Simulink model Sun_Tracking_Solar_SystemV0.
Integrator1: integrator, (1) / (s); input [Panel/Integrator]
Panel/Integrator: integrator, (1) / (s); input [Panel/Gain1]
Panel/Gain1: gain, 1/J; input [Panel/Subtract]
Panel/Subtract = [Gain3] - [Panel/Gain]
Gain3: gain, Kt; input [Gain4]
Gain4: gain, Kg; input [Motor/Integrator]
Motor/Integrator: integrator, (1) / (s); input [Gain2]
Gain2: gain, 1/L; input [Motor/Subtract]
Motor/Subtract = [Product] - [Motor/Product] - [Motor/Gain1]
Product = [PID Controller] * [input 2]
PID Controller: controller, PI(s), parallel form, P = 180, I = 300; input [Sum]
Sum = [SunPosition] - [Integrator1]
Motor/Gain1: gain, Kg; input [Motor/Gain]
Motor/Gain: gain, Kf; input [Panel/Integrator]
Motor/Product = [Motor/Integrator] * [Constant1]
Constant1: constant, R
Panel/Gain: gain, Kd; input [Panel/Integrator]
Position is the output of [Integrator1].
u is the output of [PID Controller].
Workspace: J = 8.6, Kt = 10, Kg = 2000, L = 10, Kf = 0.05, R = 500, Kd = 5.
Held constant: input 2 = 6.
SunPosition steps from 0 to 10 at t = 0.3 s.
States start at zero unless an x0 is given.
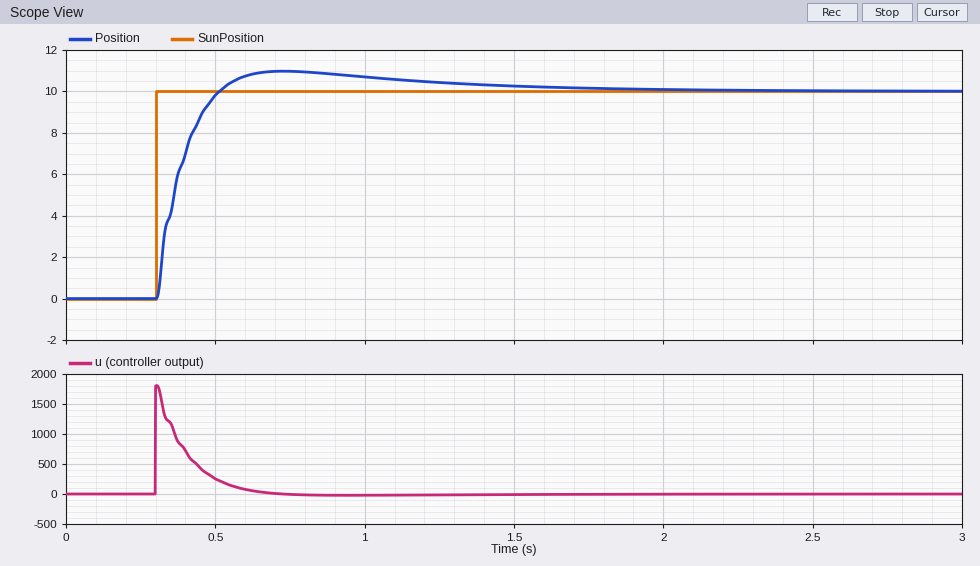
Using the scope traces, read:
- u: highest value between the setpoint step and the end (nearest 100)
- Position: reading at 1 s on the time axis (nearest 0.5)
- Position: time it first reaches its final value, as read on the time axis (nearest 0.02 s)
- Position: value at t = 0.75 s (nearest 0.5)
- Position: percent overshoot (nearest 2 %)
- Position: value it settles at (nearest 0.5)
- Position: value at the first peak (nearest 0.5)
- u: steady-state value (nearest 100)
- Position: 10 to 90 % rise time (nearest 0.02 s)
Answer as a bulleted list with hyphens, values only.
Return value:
- 1800
- 10.5
- 0.52 s
- 11.0
- 10 %
- 10.0
- 11.0
- 0
- 0.14 s
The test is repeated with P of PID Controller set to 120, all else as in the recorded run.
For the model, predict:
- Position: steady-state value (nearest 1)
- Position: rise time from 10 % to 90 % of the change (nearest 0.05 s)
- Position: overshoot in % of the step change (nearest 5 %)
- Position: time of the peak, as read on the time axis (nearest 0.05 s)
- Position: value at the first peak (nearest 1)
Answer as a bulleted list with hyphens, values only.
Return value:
- 10
- 0.20 s
- 15 %
- 0.80 s
- 12
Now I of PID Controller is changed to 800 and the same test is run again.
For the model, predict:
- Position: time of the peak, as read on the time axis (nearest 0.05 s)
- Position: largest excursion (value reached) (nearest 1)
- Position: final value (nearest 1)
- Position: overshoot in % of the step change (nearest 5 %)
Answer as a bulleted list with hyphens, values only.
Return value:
- 0.60 s
- 12
- 10
- 20 %
